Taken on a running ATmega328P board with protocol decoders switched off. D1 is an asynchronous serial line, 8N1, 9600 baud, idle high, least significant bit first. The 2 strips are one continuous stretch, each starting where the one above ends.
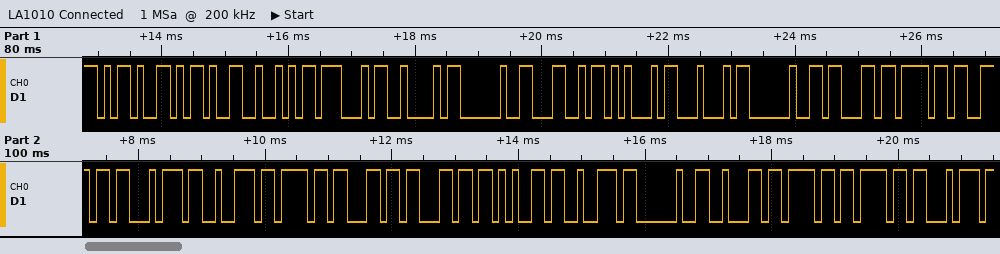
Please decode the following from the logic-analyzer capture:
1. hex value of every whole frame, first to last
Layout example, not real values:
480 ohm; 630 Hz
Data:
2D 2D 52 47 42 20 4C 45 44 20 63 6F 6E 74 72 6F 6C 6C 65 72 20 62 6F 6F 74
